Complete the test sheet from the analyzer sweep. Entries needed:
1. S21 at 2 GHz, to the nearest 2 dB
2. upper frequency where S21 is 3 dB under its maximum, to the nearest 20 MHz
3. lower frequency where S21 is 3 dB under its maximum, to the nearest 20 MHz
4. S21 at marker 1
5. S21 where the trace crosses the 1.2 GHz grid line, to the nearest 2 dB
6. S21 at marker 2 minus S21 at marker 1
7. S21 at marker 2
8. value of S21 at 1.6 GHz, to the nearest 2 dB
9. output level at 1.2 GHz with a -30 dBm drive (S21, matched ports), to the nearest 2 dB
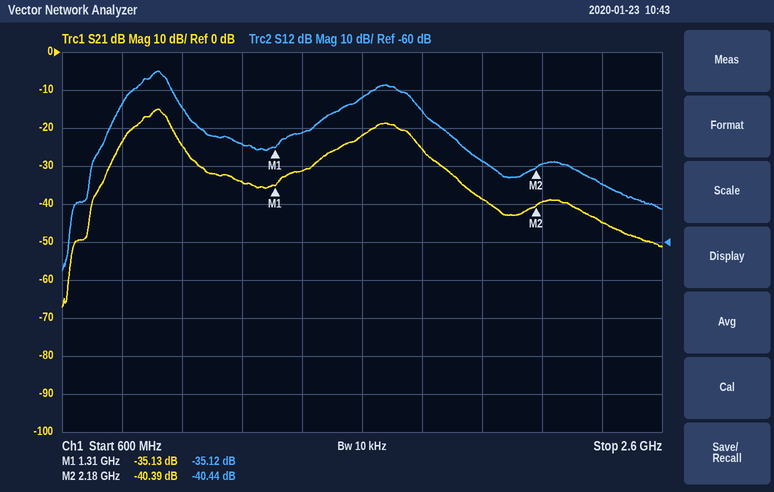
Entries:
-38 dB
960 MHz
860 MHz
-35.13 dB
-34 dB
-5.26 dB
-40.39 dB
-22 dB
-64 dBm
